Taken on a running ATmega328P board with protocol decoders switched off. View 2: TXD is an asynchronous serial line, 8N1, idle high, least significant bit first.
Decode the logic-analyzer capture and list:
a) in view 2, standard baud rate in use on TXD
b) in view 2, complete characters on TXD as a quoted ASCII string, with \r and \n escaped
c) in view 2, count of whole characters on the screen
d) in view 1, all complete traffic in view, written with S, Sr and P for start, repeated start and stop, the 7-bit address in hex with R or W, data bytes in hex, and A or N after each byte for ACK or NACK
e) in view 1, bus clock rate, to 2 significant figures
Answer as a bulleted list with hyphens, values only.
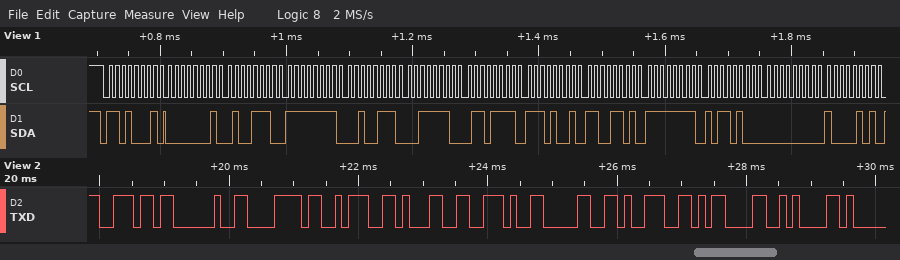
- 9600 baud
- "n x:1.09\r\n"
- 10
- S 68R A 01 A 4E A FF A 27 A 3E A 6F A E9 A CD A FF A B4 A 00 A 85 A
- 100 kHz
